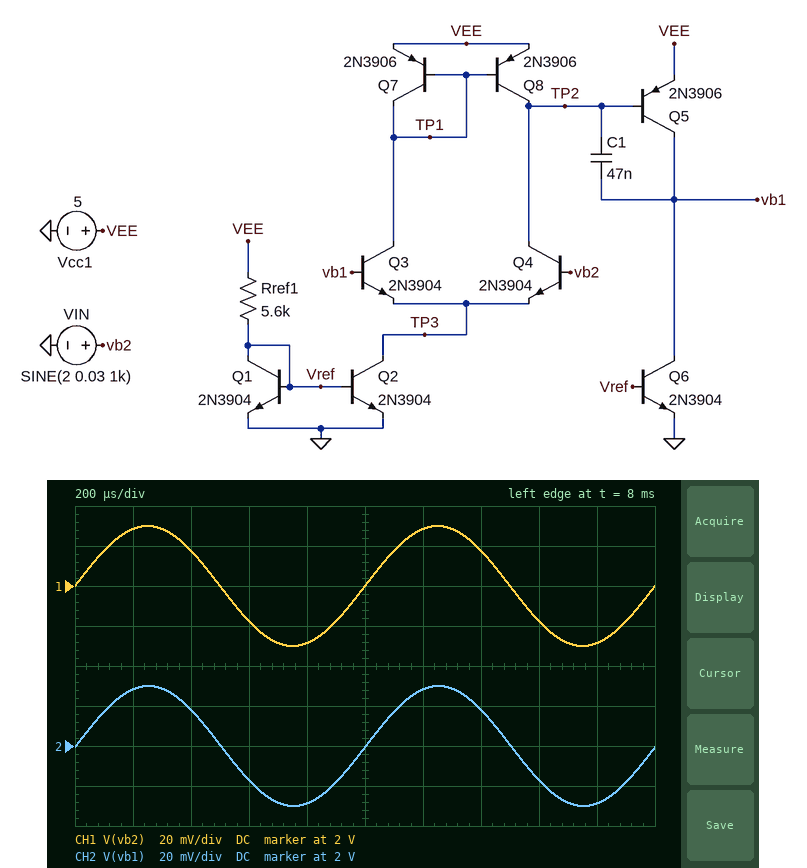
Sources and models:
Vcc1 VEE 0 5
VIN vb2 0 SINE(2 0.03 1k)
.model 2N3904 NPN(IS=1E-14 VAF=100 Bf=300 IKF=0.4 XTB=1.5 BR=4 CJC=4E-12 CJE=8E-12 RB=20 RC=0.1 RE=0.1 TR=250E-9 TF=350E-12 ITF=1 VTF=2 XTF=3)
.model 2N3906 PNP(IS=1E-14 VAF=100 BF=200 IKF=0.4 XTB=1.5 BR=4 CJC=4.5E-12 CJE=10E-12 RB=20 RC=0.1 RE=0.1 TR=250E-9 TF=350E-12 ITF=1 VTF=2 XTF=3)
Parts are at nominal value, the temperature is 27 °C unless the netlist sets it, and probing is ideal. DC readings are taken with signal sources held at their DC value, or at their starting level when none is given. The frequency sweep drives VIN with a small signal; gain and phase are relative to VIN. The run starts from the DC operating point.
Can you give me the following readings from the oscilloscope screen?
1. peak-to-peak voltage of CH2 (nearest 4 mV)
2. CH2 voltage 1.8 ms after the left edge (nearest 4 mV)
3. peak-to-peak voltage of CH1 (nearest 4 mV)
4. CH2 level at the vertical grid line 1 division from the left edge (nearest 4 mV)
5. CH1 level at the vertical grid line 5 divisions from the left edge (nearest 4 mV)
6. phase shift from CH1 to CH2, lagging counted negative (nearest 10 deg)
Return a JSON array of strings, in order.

["60 mV", "1.972 V", "60 mV", "2.028 V", "2.000 V", "0 deg"]
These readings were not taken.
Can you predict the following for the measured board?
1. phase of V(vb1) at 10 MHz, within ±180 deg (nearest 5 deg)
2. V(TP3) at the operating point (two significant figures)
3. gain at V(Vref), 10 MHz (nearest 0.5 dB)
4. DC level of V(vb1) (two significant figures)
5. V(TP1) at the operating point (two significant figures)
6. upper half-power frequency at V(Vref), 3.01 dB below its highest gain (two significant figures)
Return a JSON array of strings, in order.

["155 deg", "1.4 V", "-45.5 dB", "2.0 V", "4.4 V", "1.8 GHz"]
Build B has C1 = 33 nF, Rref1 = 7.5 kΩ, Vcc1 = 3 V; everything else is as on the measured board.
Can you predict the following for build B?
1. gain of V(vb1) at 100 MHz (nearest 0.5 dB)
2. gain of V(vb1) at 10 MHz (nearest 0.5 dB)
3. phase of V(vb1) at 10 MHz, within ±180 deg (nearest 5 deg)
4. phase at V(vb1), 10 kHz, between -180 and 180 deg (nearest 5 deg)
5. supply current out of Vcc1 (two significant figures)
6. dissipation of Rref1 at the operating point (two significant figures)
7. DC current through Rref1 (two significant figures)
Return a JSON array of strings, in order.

["-12.0 dB", "-3.5 dB", "130 deg", "-20 deg", "950 µA", "750 µW", "320 µA"]
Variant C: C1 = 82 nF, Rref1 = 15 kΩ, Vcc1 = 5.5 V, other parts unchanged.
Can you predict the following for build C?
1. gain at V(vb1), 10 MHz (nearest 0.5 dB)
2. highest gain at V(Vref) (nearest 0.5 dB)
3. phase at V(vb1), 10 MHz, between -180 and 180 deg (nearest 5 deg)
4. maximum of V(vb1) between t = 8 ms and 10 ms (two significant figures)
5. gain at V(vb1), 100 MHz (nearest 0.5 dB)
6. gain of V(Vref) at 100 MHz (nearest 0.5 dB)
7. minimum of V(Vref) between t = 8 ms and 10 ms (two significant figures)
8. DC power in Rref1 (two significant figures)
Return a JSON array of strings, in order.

["-3.0 dB", "-27.5 dB", "130 deg", "2.0 V", "-12.5 dB", "-29.0 dB", "630 mV", "1.6 mW"]
